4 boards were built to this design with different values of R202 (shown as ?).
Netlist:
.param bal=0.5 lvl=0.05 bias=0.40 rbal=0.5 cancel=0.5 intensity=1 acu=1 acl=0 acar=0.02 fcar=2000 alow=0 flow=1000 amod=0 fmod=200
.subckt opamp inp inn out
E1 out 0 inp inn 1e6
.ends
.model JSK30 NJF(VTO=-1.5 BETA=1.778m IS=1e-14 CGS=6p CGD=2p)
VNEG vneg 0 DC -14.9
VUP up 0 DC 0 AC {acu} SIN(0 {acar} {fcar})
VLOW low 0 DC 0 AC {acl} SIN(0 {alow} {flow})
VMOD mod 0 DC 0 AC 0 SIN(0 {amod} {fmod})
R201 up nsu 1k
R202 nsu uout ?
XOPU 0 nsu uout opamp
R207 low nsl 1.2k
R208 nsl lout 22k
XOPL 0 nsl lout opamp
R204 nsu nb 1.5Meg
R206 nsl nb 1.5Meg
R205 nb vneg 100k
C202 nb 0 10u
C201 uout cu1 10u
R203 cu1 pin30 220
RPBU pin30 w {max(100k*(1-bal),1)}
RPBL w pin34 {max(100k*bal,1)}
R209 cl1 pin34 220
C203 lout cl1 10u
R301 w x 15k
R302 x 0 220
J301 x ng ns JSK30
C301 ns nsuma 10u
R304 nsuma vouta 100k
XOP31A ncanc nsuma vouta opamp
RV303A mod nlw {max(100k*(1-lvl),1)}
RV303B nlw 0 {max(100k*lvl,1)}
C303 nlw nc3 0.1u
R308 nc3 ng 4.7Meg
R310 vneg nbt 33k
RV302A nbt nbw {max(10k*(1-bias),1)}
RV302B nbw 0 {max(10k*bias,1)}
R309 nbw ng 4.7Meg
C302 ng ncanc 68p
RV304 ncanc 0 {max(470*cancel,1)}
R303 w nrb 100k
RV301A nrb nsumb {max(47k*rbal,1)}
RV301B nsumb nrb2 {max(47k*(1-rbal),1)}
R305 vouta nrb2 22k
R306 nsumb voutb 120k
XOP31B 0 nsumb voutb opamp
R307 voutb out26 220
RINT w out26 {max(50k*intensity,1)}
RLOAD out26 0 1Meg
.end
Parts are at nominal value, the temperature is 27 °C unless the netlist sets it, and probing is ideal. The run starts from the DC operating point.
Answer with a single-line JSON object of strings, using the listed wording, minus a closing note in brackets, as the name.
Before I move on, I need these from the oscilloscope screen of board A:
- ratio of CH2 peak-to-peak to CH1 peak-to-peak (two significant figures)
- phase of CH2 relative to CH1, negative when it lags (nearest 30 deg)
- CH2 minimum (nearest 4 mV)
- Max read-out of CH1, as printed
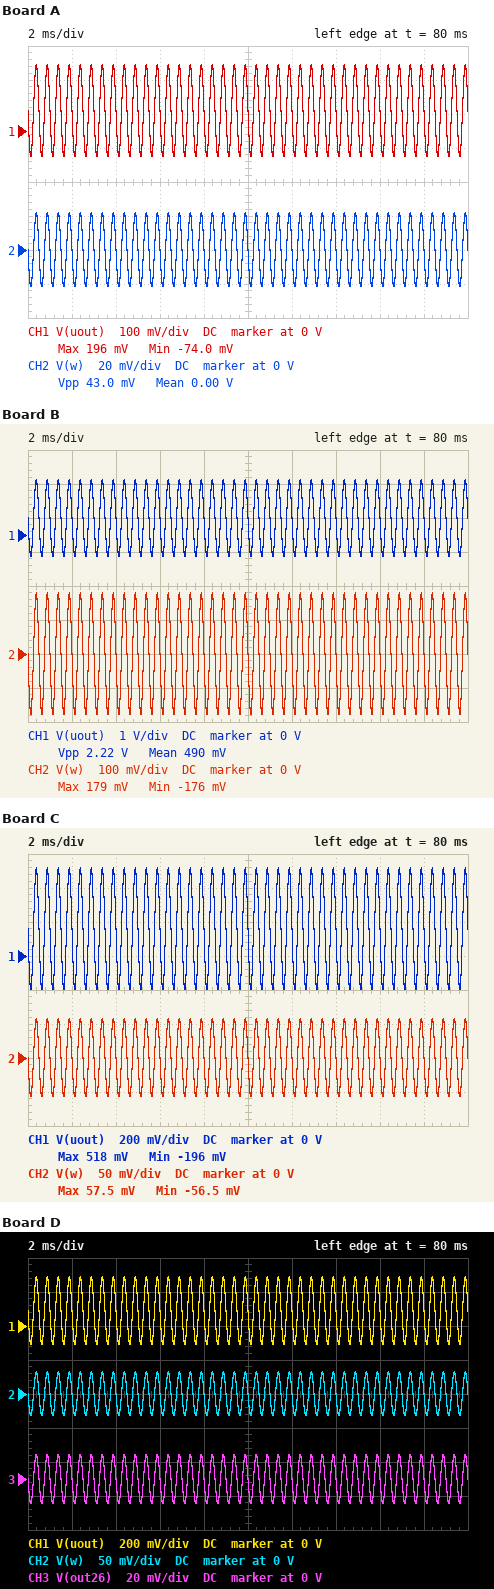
{"ratio of CH2 peak-to-peak to CH1 peak-to-peak": "0.16", "phase of CH2 relative to CH1, negative when it lags": "0 deg", "CH2 minimum": "-20 mV", "Max read-out of CH1, as printed": "196 mV"}
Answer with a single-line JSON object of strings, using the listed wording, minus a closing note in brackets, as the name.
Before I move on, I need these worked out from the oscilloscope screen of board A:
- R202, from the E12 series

{"R202, from the E12 series": "6.8 kΩ"}
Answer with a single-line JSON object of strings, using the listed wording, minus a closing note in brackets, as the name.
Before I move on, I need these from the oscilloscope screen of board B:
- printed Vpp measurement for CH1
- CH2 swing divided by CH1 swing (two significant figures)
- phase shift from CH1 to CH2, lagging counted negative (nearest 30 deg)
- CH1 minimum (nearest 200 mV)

{"printed Vpp measurement for CH1": "2.22 V", "CH2 swing divided by CH1 swing": "0.16", "phase shift from CH1 to CH2, lagging counted negative": "0 deg", "CH1 minimum": "-600 mV"}
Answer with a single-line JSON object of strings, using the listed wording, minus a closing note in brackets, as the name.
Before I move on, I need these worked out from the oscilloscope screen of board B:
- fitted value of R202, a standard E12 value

{"fitted value of R202, a standard E12 value": "56 kΩ"}
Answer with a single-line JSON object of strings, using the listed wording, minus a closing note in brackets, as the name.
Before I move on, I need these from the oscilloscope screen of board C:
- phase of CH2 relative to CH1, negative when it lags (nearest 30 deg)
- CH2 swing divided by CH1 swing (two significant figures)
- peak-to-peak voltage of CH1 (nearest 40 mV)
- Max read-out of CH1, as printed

{"phase of CH2 relative to CH1, negative when it lags": "0 deg", "CH2 swing divided by CH1 swing": "0.16", "peak-to-peak voltage of CH1": "720 mV", "Max read-out of CH1, as printed": "518 mV"}
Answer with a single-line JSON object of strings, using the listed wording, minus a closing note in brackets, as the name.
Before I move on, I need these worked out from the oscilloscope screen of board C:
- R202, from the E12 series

{"R202, from the E12 series": "18 kΩ"}
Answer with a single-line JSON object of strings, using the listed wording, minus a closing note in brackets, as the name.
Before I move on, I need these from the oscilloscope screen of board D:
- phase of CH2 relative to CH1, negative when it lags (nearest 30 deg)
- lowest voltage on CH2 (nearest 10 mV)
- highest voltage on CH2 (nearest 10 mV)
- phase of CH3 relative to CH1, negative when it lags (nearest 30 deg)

{"phase of CH2 relative to CH1, negative when it lags": "0 deg", "lowest voltage on CH2": "-30 mV", "highest voltage on CH2": "30 mV", "phase of CH3 relative to CH1, negative when it lags": "0 deg"}
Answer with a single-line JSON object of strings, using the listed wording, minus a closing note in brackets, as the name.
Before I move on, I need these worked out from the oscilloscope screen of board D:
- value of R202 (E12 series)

{"value of R202": "10 kΩ"}
